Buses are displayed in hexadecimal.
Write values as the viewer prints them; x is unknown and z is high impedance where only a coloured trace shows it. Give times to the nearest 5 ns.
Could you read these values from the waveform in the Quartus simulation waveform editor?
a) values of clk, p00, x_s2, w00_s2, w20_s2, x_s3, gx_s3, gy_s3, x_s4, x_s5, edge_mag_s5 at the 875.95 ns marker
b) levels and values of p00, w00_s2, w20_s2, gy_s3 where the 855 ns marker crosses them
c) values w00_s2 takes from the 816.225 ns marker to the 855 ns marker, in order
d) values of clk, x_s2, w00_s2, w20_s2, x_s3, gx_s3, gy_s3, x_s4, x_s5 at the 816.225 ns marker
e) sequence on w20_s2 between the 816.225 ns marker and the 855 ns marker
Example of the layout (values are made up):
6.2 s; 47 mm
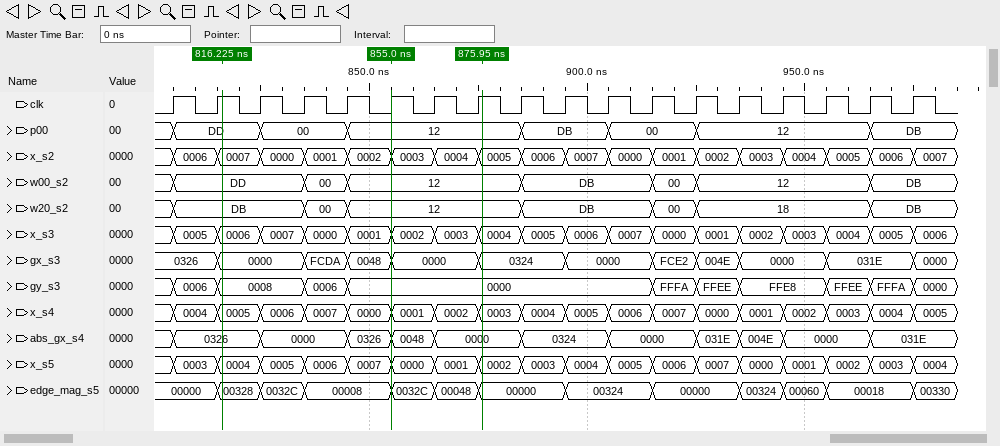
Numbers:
clk=1, p00=12, x_s2=0005, w00_s2=12, w20_s2=12, x_s3=0004, gx_s3=0324, gy_s3=0000, x_s4=0003, x_s5=0002, edge_mag_s5=00000; p00=12, w00_s2=12, w20_s2=12, gy_s3=0000; DD, 00, 12; clk=1, x_s2=0007, w00_s2=DD, w20_s2=DB, x_s3=0006, gx_s3=0000, gy_s3=0008, x_s4=0005, x_s5=0004; DB, 00, 12
